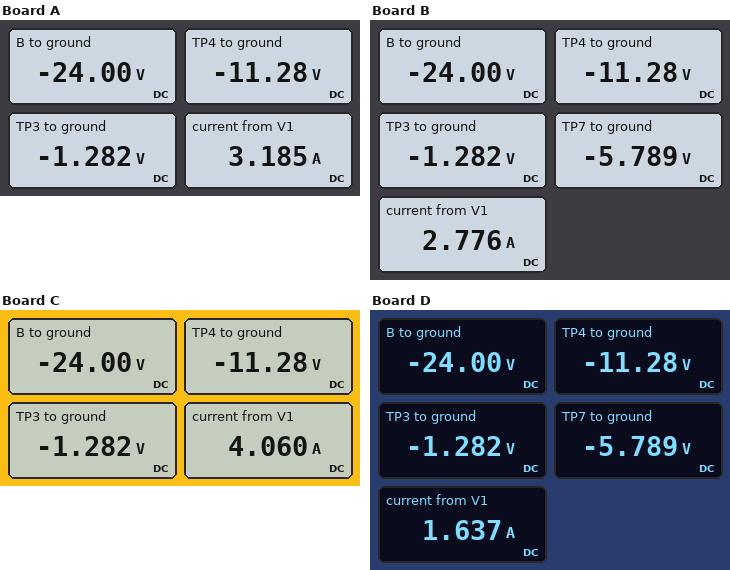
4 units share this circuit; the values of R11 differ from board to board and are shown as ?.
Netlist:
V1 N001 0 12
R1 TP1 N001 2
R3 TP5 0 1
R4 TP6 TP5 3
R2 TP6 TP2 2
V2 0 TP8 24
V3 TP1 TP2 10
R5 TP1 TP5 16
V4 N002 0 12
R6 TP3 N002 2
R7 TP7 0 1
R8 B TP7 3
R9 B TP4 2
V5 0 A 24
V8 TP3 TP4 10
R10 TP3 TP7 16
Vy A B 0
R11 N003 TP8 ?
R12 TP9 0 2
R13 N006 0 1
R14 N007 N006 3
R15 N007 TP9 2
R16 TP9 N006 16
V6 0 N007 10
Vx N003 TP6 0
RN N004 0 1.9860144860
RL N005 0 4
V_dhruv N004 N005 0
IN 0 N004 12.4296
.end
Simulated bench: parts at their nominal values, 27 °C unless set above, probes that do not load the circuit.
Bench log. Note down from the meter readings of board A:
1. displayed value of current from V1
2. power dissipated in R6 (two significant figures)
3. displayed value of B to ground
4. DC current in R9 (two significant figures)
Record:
3.185 A
88 W
-24.00 V
6.4 A
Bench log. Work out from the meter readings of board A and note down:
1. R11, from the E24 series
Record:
2.7 Ω
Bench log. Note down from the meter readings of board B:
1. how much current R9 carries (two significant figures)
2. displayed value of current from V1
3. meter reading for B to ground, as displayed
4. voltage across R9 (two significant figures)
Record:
6.4 A
2.776 A
-24.00 V
13 V
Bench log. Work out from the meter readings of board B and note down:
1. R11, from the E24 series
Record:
3.6 Ω
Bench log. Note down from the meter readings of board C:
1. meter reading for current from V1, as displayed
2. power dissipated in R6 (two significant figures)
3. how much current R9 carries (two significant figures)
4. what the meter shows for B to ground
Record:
4.060 A
88 W
6.4 A
-24.00 V
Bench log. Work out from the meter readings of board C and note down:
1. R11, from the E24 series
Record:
1.5 Ω
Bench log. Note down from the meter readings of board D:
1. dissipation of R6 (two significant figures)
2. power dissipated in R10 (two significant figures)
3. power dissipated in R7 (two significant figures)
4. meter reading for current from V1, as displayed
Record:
88 W
1.3 W
34 W
1.637 A
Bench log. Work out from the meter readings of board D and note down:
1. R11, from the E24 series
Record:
10 Ω
